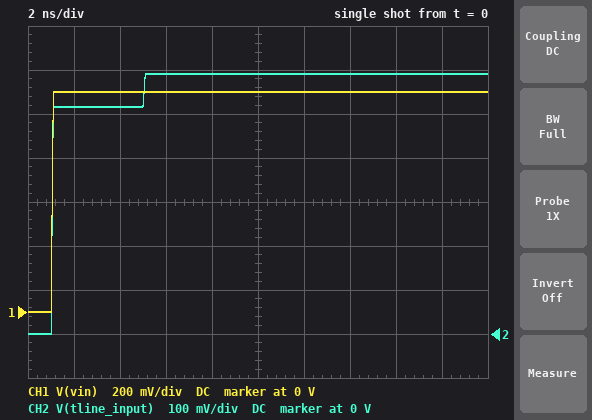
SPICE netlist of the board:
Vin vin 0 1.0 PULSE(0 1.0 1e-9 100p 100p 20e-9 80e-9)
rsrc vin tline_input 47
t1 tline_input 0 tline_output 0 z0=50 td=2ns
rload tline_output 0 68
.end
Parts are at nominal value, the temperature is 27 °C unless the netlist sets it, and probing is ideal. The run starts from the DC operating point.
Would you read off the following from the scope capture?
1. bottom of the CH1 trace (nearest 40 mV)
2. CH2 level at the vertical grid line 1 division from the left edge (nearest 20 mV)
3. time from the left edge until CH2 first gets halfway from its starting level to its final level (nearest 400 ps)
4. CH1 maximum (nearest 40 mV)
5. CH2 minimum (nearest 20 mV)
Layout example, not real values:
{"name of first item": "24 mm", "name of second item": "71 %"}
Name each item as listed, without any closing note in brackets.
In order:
{"bottom of the CH1 trace": "0 V", "CH2 level at the vertical grid line 1 division from the left edge": "520 mV", "time from the left edge until CH2 first gets halfway from its starting level to its final level": "1.2 ns", "CH1 maximum": "1.00 V", "CH2 minimum": "0 V"}
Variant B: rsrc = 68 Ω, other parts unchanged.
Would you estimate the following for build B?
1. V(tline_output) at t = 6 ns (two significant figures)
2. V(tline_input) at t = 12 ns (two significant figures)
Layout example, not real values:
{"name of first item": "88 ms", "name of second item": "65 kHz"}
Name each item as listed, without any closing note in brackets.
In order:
{"V(tline_output) at t = 6 ns": "490 mV", "V(tline_input) at t = 12 ns": "500 mV"}
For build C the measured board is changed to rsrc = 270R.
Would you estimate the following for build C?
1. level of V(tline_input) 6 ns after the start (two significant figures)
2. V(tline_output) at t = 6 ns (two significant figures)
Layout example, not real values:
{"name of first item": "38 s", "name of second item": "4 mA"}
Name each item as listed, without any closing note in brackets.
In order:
{"level of V(tline_input) 6 ns after the start": "200 mV", "V(tline_output) at t = 6 ns": "180 mV"}
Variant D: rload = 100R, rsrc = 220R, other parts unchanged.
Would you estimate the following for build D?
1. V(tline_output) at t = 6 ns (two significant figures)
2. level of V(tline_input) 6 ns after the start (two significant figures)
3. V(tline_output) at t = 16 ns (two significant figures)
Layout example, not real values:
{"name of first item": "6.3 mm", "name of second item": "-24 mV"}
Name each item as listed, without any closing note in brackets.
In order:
{"V(tline_output) at t = 6 ns": "250 mV", "level of V(tline_input) 6 ns after the start": "290 mV", "V(tline_output) at t = 16 ns": "310 mV"}
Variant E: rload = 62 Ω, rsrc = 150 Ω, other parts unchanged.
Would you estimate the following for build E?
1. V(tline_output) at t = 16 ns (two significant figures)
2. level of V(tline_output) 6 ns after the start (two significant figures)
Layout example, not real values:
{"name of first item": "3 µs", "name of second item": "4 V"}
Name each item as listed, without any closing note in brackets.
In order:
{"V(tline_output) at t = 16 ns": "290 mV", "level of V(tline_output) 6 ns after the start": "280 mV"}
